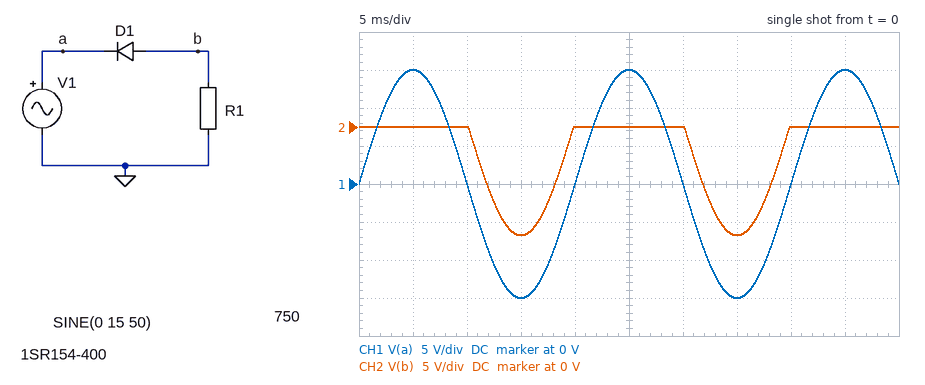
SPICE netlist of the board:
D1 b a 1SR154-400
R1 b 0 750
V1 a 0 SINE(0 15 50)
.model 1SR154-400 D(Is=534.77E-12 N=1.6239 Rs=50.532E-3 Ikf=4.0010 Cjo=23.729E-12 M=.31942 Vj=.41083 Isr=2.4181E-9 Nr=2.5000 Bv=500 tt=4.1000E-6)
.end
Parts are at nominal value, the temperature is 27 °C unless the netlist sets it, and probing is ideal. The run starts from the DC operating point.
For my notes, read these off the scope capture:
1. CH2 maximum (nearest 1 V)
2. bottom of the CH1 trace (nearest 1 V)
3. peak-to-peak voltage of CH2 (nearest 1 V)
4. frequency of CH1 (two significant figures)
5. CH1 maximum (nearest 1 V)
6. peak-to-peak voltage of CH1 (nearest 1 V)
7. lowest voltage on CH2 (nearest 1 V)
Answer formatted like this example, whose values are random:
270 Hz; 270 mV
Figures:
0 V; -15 V; 14 V; 50 Hz; 15 V; 30 V; -14 V
